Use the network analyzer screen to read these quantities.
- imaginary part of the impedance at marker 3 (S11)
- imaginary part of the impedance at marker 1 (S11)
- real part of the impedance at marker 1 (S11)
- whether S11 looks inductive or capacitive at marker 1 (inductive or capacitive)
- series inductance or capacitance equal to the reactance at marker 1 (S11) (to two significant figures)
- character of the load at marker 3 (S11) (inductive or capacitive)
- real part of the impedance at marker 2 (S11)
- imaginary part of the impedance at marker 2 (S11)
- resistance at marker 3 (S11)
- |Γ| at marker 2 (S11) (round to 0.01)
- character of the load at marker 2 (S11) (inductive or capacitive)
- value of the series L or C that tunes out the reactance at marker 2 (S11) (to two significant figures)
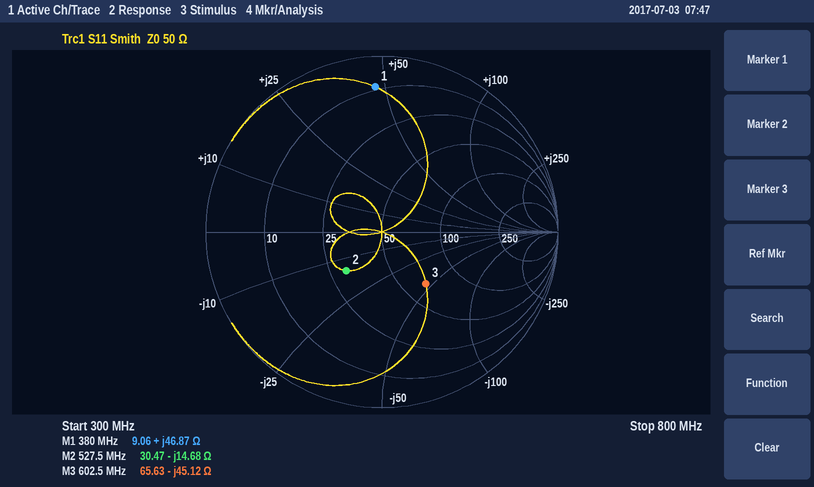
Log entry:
-45.12 Ω
+46.87 Ω
9.06 Ω
inductive
20 nH
capacitive
30.47 Ω
-14.68 Ω
65.63 Ω
0.30
capacitive
4.4 nH
